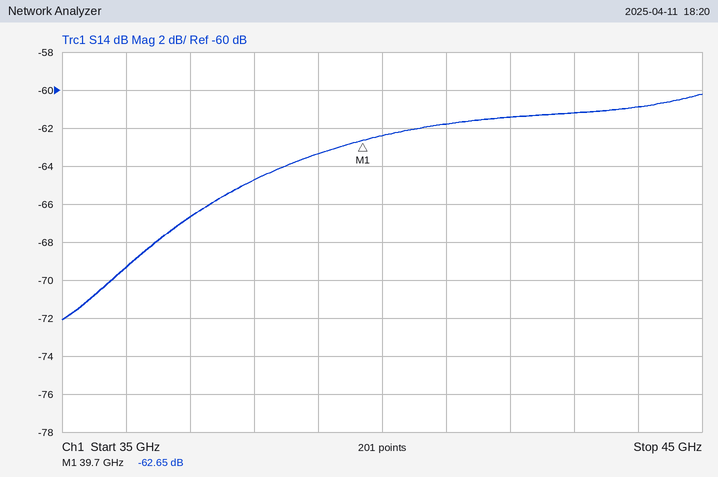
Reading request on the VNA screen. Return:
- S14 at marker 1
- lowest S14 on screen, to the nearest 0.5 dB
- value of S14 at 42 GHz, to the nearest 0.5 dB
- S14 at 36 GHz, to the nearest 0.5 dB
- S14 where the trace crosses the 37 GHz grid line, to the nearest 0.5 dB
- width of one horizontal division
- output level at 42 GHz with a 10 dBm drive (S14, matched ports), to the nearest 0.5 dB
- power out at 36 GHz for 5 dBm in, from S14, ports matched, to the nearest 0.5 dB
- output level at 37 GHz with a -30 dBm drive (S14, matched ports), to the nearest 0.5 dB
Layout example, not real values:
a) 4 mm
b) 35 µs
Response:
a) -62.65 dB
b) -72.0 dB
c) -61.5 dB
d) -69.5 dB
e) -66.5 dB
f) 1 GHz
g) -51.5 dBm
h) -64.5 dBm
i) -96.5 dBm
